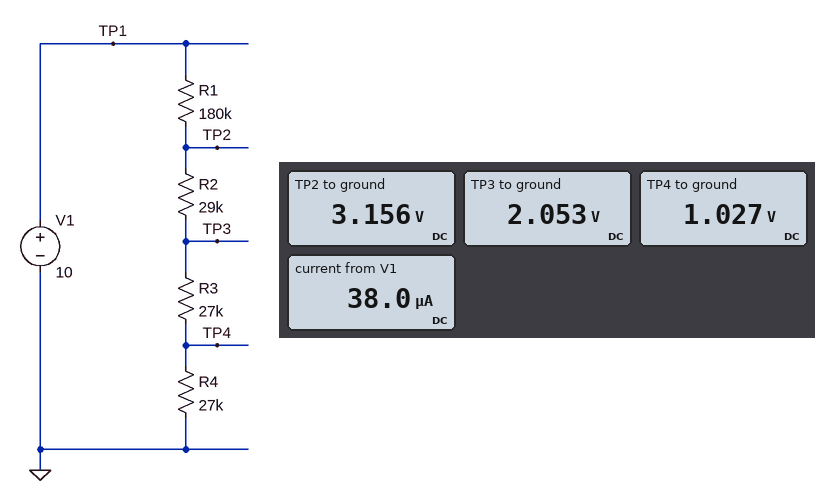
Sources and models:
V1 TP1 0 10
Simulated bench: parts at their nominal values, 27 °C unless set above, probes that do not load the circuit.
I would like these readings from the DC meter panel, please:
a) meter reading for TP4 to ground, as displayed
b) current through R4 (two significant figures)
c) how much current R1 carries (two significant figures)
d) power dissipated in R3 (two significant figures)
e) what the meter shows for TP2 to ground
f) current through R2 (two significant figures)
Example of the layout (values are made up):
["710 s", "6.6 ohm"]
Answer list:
["1.027 V", "38 µA", "38 µA", "39 µW", "3.156 V", "38 µA"]
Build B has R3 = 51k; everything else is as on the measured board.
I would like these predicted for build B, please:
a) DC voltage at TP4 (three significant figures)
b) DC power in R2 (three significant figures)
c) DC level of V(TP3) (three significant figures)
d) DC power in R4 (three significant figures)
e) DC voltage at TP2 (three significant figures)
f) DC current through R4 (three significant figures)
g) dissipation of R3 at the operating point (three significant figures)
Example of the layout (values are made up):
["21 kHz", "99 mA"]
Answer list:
["941 mV", "35.2 µW", "2.72 V", "32.8 µW", "3.73 V", "34.8 µA", "61.9 µW"]
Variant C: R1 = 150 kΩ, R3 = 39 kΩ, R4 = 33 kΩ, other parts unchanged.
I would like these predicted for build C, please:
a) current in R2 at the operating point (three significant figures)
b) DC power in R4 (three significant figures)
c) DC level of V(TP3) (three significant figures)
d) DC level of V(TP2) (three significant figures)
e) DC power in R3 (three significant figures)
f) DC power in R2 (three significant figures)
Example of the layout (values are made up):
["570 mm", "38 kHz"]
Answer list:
["39.8 µA", "52.4 µW", "2.87 V", "4.02 V", "61.9 µW", "46.0 µW"]
